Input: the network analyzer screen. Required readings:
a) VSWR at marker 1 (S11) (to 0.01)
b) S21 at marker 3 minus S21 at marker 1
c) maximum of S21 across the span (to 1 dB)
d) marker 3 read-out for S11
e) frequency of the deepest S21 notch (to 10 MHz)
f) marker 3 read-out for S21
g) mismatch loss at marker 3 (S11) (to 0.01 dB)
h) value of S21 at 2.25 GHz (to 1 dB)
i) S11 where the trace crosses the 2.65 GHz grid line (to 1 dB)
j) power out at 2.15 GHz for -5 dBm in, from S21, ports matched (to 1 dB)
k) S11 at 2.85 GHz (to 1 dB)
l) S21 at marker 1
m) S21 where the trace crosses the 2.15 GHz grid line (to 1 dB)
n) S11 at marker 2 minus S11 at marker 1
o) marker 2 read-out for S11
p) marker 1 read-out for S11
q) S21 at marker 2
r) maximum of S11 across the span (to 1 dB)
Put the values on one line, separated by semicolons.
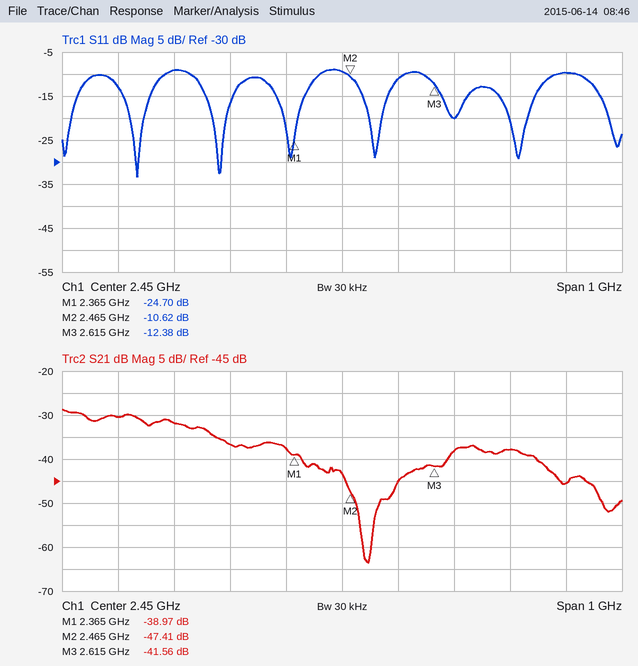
1.12; -2.59 dB; -29 dB; -12.38 dB; 2.50 GHz; -41.56 dB; 0.26 dB; -37 dB; -20 dB; -37 dBm; -10 dB; -38.97 dB; -32 dB; 14.08 dB; -10.62 dB; -24.70 dB; -47.41 dB; -9 dB
